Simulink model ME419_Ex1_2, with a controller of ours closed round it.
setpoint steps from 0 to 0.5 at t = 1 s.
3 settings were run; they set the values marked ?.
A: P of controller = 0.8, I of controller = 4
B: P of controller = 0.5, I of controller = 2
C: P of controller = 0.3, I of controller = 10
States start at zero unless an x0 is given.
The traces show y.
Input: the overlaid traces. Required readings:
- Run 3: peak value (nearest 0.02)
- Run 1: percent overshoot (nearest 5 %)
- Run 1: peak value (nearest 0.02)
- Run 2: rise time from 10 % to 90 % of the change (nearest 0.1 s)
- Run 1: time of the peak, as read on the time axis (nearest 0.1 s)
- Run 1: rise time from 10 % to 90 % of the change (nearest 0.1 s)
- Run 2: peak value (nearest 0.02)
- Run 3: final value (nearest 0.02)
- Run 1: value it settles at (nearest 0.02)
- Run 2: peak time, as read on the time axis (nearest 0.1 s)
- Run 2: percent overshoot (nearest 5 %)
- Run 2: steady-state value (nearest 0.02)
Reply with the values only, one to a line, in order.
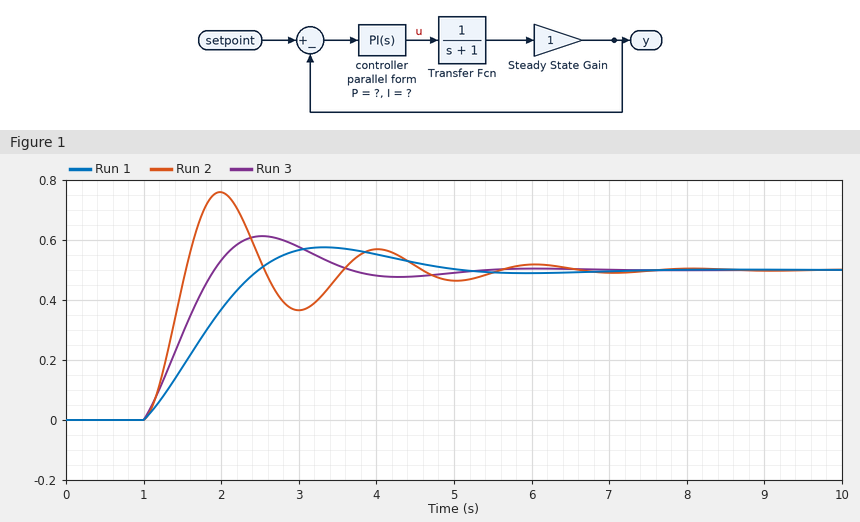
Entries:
0.62
15 %
0.58
0.4 s
3.3 s
1.1 s
0.76
0.50
0.50
2.0 s
50 %
0.50
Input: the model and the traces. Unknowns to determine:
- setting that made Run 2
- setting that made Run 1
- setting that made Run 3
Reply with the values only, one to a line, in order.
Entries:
C
B
A
